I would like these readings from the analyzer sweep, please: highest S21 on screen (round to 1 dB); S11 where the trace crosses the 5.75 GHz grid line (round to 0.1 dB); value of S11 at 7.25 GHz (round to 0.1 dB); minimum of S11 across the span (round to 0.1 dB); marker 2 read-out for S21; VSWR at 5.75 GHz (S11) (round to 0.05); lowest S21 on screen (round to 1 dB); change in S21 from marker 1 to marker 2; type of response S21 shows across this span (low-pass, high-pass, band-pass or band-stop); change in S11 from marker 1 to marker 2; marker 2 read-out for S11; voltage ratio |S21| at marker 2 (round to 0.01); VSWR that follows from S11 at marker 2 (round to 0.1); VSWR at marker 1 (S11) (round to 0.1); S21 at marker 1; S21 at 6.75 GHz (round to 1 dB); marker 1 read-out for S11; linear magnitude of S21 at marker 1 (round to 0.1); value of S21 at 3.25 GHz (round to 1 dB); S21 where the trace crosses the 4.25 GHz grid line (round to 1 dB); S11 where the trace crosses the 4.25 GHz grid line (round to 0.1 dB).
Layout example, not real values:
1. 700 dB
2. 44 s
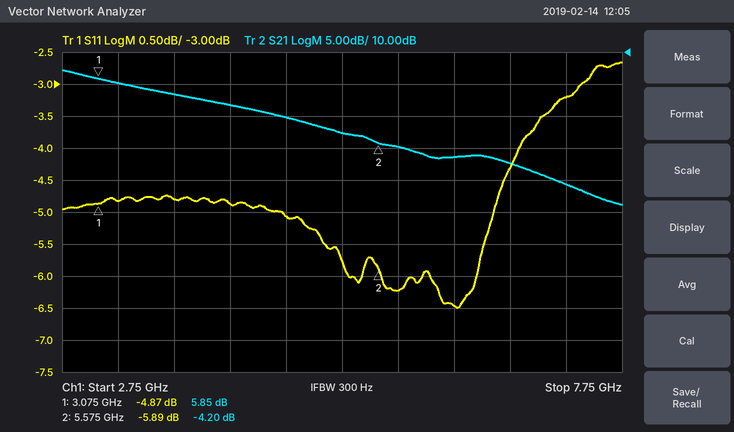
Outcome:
1. 7 dB
2. -6.2 dB
3. -3.2 dB
4. -6.5 dB
5. -4.20 dB
6. 2.90
7. -14 dB
8. -10.05 dB
9. low-pass
10. -1.02 dB
11. -5.89 dB
12. 0.62
13. 3.1
14. 3.7
15. 5.85 dB
16. -7 dB
17. -4.87 dB
18. 2.0
19. 5 dB
20. 2 dB
21. -4.9 dB
